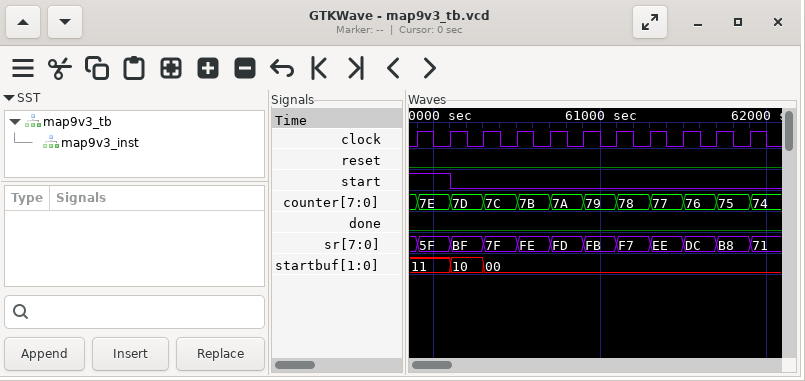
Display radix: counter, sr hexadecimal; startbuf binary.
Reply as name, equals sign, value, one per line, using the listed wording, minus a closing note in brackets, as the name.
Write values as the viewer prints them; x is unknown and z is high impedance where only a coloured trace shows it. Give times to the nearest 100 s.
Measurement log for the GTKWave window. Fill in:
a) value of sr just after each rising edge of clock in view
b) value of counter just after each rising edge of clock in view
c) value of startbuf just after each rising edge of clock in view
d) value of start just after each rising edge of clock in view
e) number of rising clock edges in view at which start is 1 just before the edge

value of sr just after each rising edge of clock in view = 5F, BF, 7F, FE, FD, FB, F7, EE, DC, B8, 71
value of counter just after each rising edge of clock in view = 7E, 7D, 7C, 7B, 7A, 79, 78, 77, 76, 75, 74
value of startbuf just after each rising edge of clock in view = 11, 10, 00, 00, 00, 00, 00, 00, 00, 00, 00
value of start just after each rising edge of clock in view = 1 0 0 0 0 0 0 0 0 0 0
number of rising clock edges in view at which start is 1 just before the edge = 2
